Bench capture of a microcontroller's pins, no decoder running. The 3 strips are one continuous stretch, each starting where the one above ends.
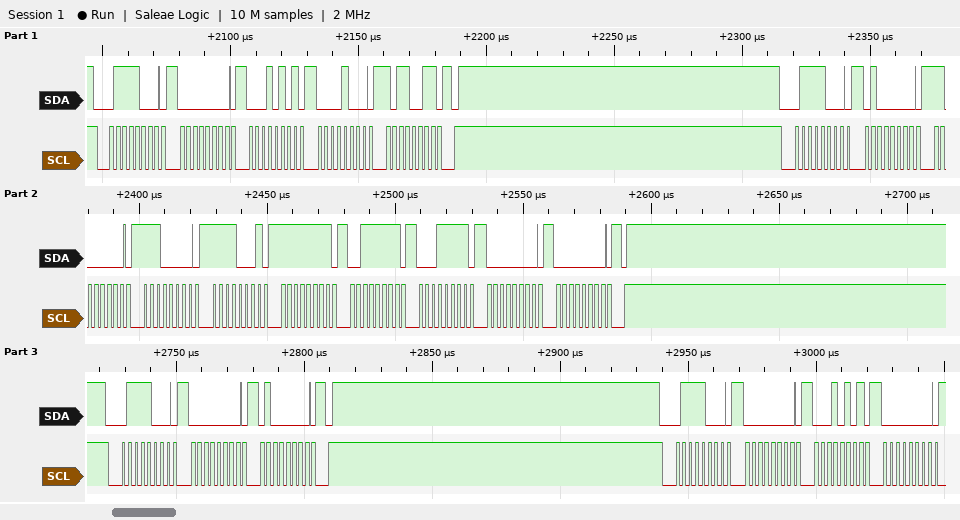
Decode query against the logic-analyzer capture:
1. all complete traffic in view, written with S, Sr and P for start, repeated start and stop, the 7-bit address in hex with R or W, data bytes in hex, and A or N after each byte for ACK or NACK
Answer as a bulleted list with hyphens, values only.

- S 3CW A 00 A 15 A 08 A B3 A P S 3CW A 40 A C0 A E0 A F1 A FF A 3F A 1F A 00 A 00 A P S 3CW A 00 A 40 A P S 3CW A 00 A 15 A 00 A
